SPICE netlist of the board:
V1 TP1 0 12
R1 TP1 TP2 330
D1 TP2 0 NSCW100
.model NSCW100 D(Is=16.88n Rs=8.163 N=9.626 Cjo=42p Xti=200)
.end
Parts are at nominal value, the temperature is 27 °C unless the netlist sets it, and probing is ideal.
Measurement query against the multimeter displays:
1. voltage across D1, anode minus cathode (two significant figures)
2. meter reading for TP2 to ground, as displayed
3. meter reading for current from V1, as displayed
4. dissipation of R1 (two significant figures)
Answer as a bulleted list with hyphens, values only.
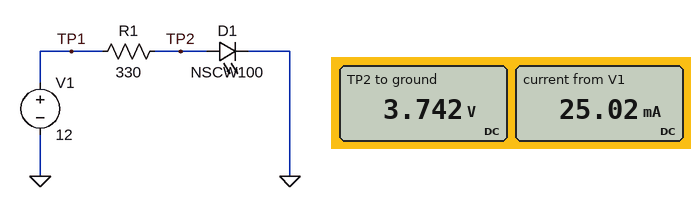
- 3.7 V
- 3.742 V
- 25.02 mA
- 210 mW
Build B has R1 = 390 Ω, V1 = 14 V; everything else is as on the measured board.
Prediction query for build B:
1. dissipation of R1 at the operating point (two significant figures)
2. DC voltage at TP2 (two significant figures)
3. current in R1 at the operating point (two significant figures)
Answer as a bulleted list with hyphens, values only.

- 270 mW
- 3.8 V
- 26 mA
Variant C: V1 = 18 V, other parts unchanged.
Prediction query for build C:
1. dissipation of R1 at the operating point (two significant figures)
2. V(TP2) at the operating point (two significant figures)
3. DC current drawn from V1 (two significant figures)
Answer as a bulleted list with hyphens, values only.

- 590 mW
- 4.0 V
- 42 mA
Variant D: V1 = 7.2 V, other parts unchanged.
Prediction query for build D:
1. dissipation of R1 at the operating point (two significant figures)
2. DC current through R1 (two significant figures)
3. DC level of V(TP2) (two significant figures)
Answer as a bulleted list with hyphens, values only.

- 43 mW
- 11 mA
- 3.4 V
